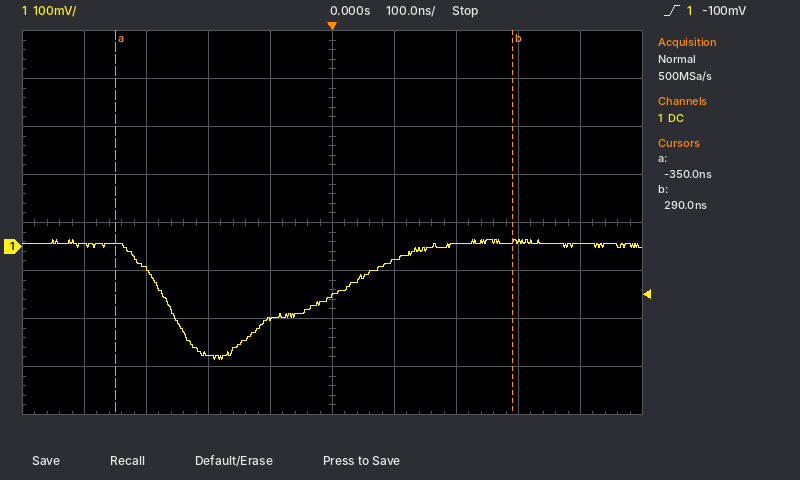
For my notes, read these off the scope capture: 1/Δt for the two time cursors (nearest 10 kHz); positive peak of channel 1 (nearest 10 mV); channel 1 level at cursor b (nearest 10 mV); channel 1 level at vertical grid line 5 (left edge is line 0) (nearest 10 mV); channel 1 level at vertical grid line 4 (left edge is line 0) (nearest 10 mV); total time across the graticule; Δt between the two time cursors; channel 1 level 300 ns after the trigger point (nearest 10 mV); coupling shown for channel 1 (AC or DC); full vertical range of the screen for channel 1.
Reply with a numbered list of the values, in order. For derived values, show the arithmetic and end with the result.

1. 1 / 640 ns ≈ 1.56 MHz
2. 10 mV
3. 10 mV
4. -100 mV
5. -150 mV
6. 1 µs
7. 290 ns − (-350 ns) = 640 ns
8. 10 mV
9. DC
10. 800 mV
